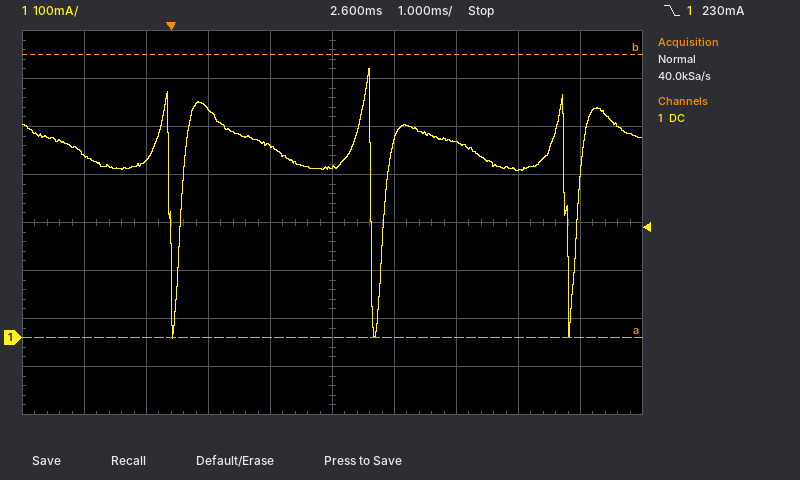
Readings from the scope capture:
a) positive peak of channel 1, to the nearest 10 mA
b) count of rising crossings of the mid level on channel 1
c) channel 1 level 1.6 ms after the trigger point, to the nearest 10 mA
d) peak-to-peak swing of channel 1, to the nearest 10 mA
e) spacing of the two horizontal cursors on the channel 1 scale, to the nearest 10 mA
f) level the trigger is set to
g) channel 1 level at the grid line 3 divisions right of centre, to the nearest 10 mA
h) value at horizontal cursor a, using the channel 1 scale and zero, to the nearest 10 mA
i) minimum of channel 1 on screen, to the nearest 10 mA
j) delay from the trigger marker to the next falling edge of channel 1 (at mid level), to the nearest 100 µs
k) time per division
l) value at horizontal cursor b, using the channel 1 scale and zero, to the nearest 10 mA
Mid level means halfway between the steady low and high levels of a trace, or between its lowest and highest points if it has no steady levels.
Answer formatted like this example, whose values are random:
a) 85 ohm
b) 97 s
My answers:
a) 560 mA
b) 3
c) 400 mA
d) 560 mA
e) 590 mA
f) 230 mA
g) 350 mA
h) 0 mA
i) 0 mA
j) 3.2 ms
k) 1 ms
l) 590 mA
